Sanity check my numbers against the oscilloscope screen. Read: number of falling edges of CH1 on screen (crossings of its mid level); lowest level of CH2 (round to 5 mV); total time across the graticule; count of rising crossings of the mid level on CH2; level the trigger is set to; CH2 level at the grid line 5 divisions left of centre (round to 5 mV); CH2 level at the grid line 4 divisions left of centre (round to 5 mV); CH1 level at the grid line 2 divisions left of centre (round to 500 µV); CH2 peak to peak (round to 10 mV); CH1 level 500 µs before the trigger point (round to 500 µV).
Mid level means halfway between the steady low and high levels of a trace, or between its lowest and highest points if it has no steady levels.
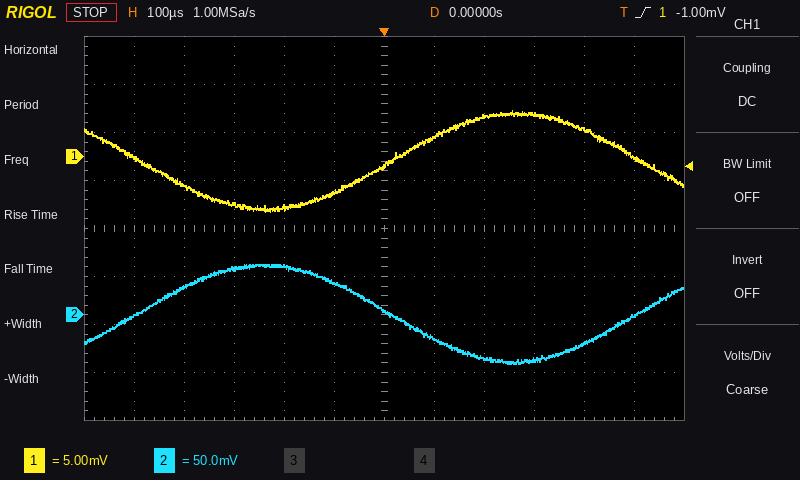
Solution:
2
-50 mV
1.2 ms
2
-1.00 mV
0 mV
30 mV
-5.5 mV
100 mV
0.0 mV
